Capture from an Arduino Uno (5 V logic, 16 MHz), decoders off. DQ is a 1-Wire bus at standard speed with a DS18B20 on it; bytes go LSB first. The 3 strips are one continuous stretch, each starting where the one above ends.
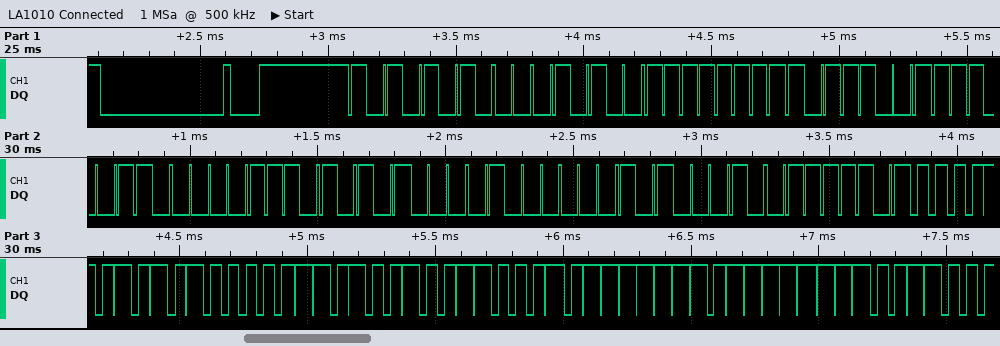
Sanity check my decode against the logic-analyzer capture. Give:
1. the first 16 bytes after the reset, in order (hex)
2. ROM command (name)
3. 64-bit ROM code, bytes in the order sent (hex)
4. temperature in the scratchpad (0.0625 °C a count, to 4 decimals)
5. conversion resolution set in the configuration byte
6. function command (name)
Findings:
55 28 FF 9D 67 70 15 02 45 BE 50 05 4B 46 7F FF
Match ROM
28 FF 9D 67 70 15 02 45
85.0000 °C
12 bits
Read Scratchpad
